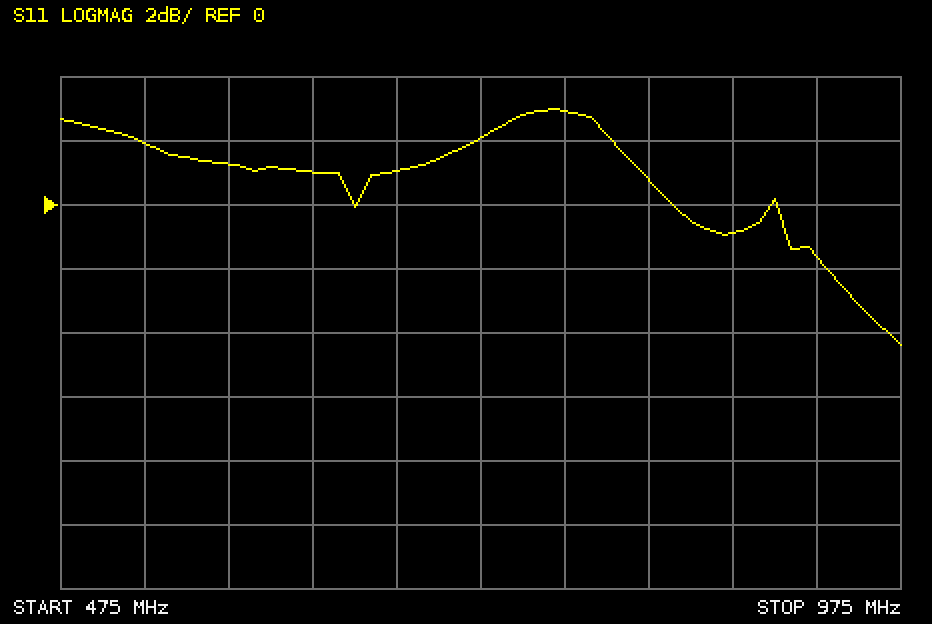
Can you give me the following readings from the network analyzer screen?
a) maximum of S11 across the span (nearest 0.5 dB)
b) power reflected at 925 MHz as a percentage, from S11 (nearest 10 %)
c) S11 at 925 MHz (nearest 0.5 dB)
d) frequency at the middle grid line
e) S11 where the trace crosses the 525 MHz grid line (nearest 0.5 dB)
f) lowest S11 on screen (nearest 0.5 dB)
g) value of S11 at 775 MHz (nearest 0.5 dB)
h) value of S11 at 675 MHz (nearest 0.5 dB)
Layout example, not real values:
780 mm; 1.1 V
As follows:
3.0 dB; 70 %; -1.5 dB; 725 MHz; 2.0 dB; -4.5 dB; 3.0 dB; 1.0 dB
